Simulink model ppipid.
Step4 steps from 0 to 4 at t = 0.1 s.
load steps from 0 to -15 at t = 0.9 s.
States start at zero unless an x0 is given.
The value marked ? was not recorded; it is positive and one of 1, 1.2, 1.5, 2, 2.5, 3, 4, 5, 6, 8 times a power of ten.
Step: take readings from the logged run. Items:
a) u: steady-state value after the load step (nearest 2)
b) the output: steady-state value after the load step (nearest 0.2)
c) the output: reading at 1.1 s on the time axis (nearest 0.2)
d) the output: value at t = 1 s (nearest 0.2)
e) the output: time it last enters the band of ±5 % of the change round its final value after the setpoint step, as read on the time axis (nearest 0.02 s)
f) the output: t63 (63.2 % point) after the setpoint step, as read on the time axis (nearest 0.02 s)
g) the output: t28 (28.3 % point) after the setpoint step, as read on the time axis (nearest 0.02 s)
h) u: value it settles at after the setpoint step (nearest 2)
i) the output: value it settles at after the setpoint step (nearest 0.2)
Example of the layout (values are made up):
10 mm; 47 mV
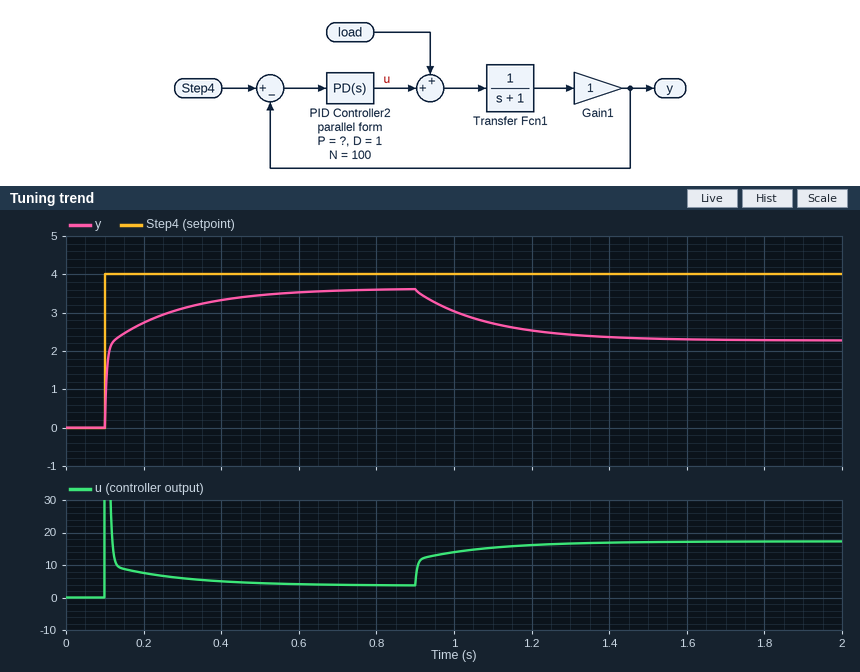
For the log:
18; 2.2; 2.8; 3.0; 0.50 s; 0.12 s; 0.10 s; 4; 3.6
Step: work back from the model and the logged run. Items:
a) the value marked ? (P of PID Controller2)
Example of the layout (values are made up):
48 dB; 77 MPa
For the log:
10
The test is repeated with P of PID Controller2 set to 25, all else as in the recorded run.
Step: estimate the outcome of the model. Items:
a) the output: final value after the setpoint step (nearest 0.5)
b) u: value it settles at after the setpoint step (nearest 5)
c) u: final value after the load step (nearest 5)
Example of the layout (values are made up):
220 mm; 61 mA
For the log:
4.0; 5; 20
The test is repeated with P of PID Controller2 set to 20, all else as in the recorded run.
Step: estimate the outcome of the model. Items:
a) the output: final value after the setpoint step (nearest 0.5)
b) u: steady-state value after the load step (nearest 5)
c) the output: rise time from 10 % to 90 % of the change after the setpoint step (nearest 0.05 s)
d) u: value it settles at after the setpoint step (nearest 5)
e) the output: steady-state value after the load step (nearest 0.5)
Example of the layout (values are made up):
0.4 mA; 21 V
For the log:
4.0; 20; 0.15 s; 5; 3.0
